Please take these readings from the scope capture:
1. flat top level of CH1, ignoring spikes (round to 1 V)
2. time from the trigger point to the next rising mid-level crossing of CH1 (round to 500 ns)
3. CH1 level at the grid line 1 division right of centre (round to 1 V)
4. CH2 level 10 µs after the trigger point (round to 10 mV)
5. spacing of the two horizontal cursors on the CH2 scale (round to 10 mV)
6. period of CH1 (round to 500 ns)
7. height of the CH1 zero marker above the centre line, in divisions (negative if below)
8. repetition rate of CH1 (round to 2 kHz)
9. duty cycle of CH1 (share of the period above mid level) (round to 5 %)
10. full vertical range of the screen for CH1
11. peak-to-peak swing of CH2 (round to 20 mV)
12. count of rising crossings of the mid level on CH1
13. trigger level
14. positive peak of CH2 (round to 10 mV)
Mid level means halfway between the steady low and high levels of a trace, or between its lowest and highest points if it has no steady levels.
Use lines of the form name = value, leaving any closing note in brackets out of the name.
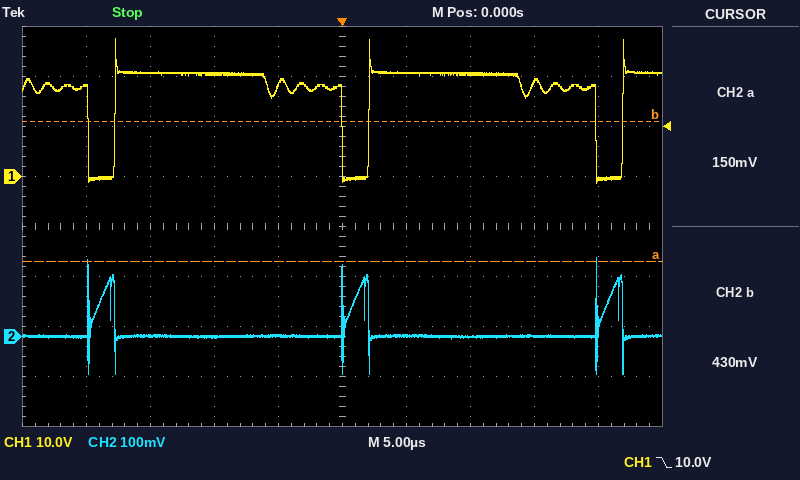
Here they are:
flat top level of CH1, ignoring spikes = 21 V
time from the trigger point to the next rising mid-level crossing of CH1 = 2.0 µs
CH1 level at the grid line 1 division right of centre = 21 V
CH2 level 10 µs after the trigger point = 0 mV
spacing of the two horizontal cursors on the CH2 scale = 280 mV
period of CH1 = 20.0 µs
height of the CH1 zero marker above the centre line, in divisions = +1.0 div
repetition rate of CH1 = 50 kHz
duty cycle of CH1 (share of the period above mid level) = 90 %
full vertical range of the screen for CH1 = 80 V
peak-to-peak swing of CH2 = 240 mV
count of rising crossings of the mid level on CH1 = 3
trigger level = 10.0 V
positive peak of CH2 = 160 mV
